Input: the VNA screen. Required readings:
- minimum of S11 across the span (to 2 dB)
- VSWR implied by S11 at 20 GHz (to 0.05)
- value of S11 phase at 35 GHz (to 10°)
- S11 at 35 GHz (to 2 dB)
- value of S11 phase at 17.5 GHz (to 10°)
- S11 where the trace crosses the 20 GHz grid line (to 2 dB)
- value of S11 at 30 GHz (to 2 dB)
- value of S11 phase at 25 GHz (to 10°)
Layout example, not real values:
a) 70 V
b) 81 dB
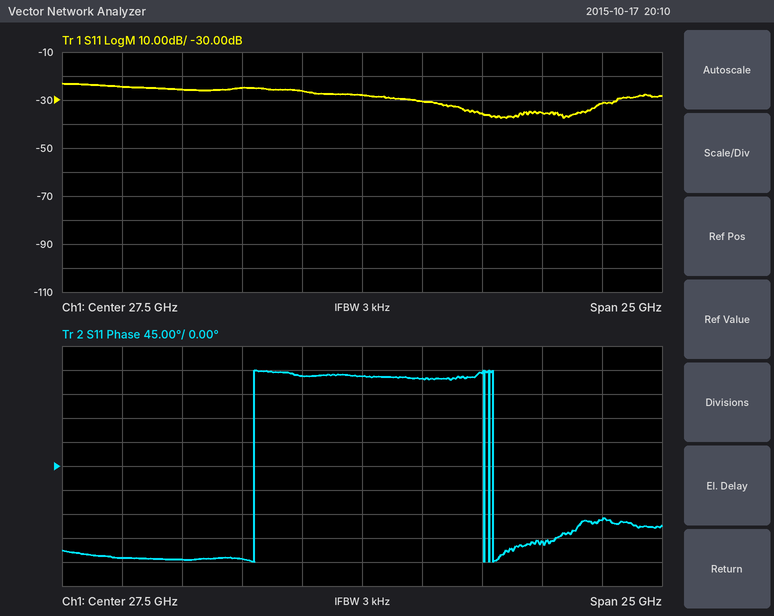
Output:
a) -38 dB
b) 1.10
c) -140°
d) -36 dB
e) -170°
f) -26 dB
g) -30 dB
h) 170°
